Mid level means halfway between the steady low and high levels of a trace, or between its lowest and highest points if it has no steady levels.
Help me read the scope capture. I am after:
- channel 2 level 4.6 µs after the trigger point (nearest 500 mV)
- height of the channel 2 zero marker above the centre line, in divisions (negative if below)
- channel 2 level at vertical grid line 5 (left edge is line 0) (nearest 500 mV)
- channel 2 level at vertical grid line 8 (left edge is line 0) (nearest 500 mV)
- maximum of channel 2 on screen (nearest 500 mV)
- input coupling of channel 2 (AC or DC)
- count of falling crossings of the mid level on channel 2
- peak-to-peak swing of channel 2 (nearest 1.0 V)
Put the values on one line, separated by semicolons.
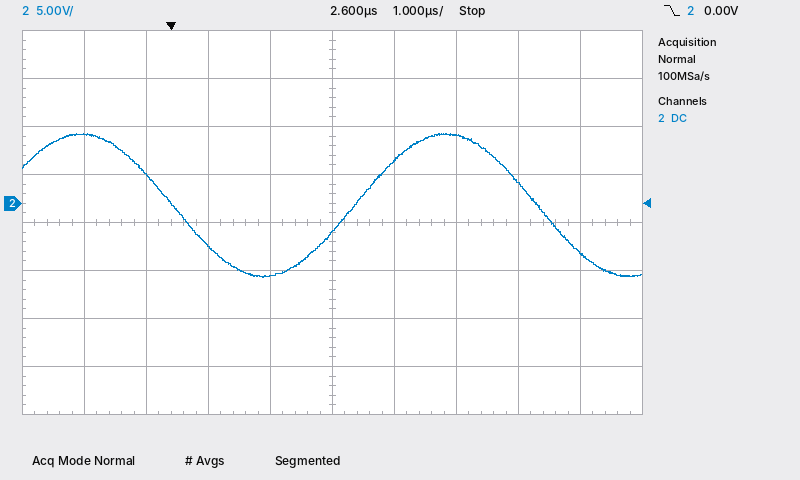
7.0 V; +0.4 div; -3.0 V; 2.0 V; 7.5 V; DC; 2; 15.0 V
